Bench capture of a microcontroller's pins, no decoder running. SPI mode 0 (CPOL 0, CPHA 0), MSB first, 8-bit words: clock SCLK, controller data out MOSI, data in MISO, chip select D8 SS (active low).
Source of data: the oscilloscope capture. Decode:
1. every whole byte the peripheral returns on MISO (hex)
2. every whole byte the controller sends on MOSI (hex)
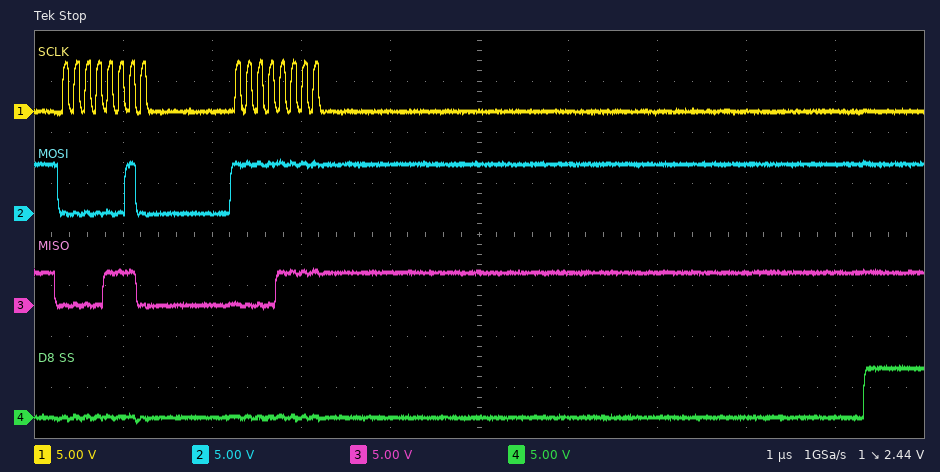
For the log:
0E 0F
02 FF
